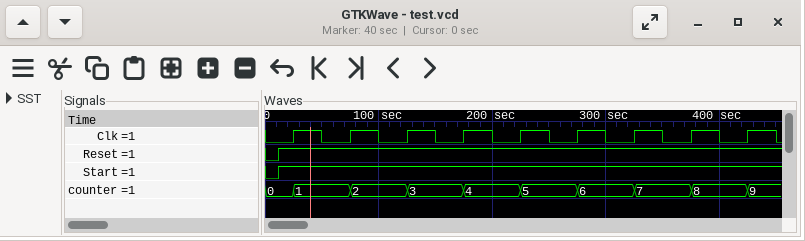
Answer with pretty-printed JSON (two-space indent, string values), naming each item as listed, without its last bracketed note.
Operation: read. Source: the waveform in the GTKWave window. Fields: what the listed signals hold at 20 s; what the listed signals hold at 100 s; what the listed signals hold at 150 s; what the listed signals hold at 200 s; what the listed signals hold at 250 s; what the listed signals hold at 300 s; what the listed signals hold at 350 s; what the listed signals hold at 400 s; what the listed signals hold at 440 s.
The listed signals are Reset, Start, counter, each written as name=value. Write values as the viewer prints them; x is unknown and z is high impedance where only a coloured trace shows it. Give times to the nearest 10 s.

{
  "what the listed signals hold at 20 s": "Reset=1, Start=1, counter=0",
  "what the listed signals hold at 100 s": "Reset=1, Start=1, counter=2",
  "what the listed signals hold at 150 s": "Reset=1, Start=1, counter=3",
  "what the listed signals hold at 200 s": "Reset=1, Start=1, counter=4",
  "what the listed signals hold at 250 s": "Reset=1, Start=1, counter=5",
  "what the listed signals hold at 300 s": "Reset=1, Start=1, counter=6",
  "what the listed signals hold at 350 s": "Reset=1, Start=1, counter=7",
  "what the listed signals hold at 400 s": "Reset=1, Start=1, counter=8",
  "what the listed signals hold at 440 s": "Reset=1, Start=1, counter=9"
}
